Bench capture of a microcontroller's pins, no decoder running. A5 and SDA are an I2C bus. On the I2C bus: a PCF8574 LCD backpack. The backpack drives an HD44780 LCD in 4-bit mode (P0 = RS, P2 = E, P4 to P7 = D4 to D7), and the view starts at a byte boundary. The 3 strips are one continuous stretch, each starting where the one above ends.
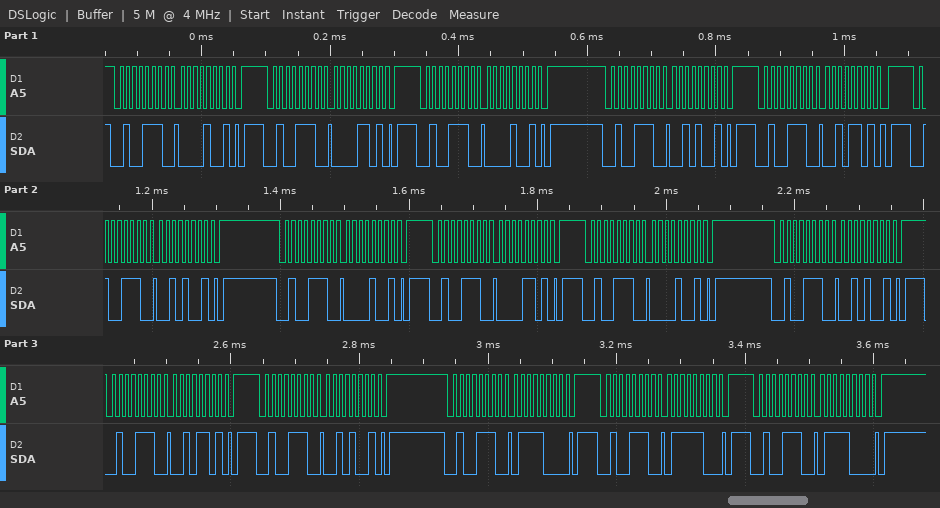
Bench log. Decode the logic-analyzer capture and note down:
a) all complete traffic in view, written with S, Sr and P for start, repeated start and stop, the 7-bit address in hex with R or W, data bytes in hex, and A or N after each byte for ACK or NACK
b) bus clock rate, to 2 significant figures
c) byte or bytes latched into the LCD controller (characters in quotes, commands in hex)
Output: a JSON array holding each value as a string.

["S 27W A 09 A P S 27W A 0D A P S 27W A 09 A P S 27W A 29 A P S 27W A 2D A P S 27W A 29 A P S 27W A 09 A P S 27W A 0D A P S 27W A 09 A P S 27W A 29 A P S 27W A 2D A P S 27W A 29 A P S 27W A 78 A P S 27W A 7C A P S 27W A 78 A P", "100 kHz", "data 0x02 data 0x02"]
